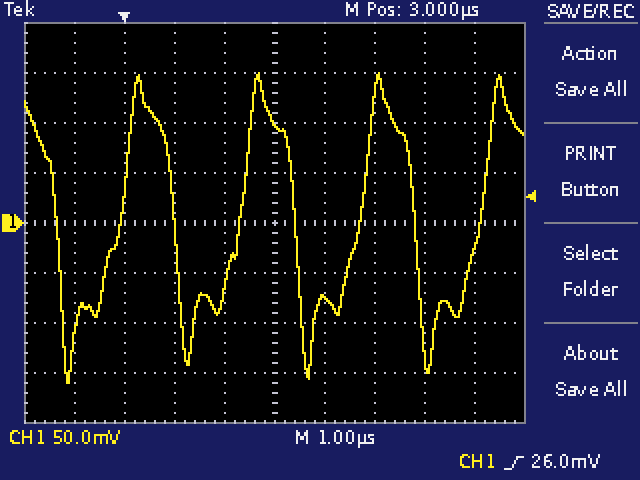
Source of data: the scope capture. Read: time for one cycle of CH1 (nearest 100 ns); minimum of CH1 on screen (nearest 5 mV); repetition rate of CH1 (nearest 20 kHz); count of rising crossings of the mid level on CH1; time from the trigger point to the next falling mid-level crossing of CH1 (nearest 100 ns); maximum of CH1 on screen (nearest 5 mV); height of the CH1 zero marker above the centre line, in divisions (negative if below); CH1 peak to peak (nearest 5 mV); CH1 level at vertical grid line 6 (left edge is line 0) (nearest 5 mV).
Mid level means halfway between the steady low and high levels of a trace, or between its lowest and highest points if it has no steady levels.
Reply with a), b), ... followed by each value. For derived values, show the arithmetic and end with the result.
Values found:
a) 2.4 µs
b) -160 mV
c) 1 / 2.4 µs ≈ 417 kHz, so 420 kHz to the nearest 20 kHz
d) 4
e) 1.0 µs
f) 150 mV
g) 0.0 div
h) 150 mV − (-160 mV) = 310 mV
i) -75 mV
